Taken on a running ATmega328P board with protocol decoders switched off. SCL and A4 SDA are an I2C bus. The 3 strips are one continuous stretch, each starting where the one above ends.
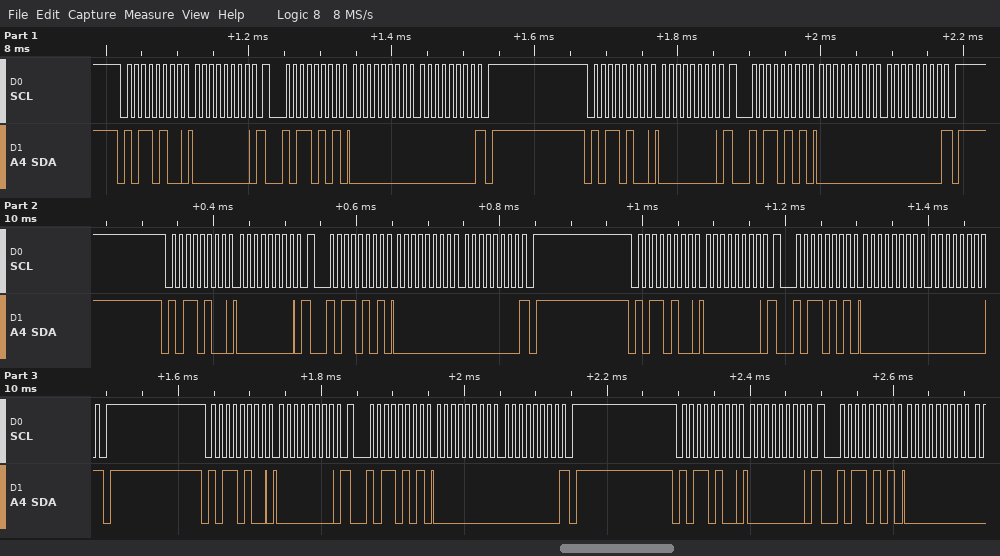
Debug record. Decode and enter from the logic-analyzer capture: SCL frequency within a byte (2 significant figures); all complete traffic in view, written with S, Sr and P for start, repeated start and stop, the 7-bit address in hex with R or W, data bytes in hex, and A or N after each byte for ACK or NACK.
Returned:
100 kHz
S 5AW A 00 A Sr 5AR A 00 A 00 N P S 5AW A 00 A Sr 5AR A 00 A 00 N P S 5AW A 00 A Sr 5AR A 00 A 00 N P S 5AW A 00 A Sr 5AR A 00 A 00 N P S 5AW A 00 A Sr 5AR A 00 A 00 N P S 5AW A 00 A Sr 5AR A 00 A
